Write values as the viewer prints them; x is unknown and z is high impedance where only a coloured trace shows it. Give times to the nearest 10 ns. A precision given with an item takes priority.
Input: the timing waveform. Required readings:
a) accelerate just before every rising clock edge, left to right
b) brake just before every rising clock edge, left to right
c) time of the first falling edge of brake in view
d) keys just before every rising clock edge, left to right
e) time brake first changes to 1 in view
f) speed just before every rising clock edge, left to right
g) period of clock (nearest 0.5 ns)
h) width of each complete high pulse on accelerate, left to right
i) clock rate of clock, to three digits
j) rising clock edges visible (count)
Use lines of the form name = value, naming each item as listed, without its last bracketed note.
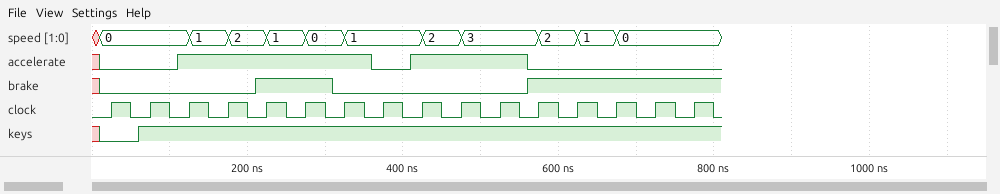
accelerate just before every rising clock edge, left to right = 0 0 1 1 1 1 1 0 1 1 1 0 0 0 0 0
brake just before every rising clock edge, left to right = 0 0 0 0 1 1 0 0 0 0 0 1 1 1 1 1
time of the first falling edge of brake in view = 310 ns
keys just before every rising clock edge, left to right = 0 1 1 1 1 1 1 1 1 1 1 1 1 1 1 1
time brake first changes to 1 in view = 210 ns
speed just before every rising clock edge, left to right = 0, 0, 0, 1, 2, 1, 0, 1, 1, 2, 3, 3, 2, 1, 0, 0
period of clock = 50 ns
width of each complete high pulse on accelerate, left to right = 250 ns, 150 ns
clock rate of clock, to three digits = 20.0 MHz
rising clock edges visible = 16
